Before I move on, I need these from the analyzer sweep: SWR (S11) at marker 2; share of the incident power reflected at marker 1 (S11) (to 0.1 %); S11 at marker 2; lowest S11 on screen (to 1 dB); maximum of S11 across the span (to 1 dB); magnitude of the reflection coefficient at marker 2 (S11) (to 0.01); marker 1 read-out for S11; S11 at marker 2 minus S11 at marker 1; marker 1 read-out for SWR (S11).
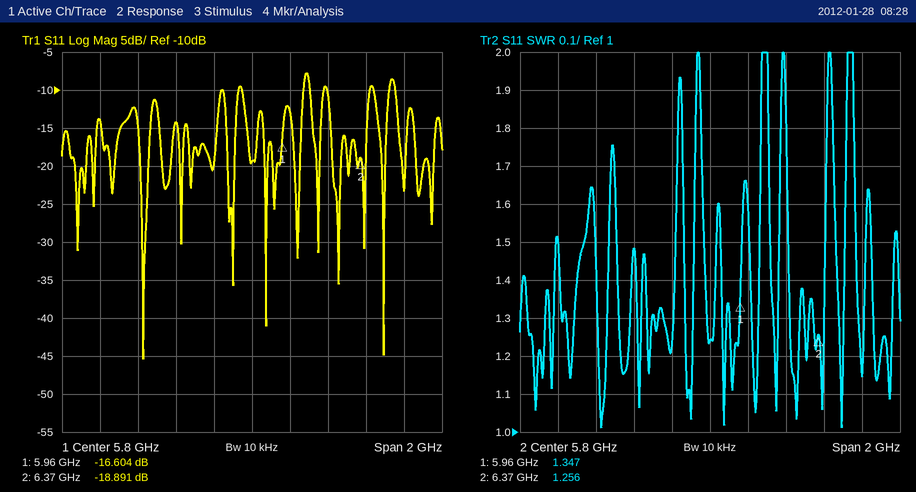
1.256
2.2 %
-18.891 dB
-45 dB
-8 dB
0.11
-16.604 dB
-2.287 dB
1.347
